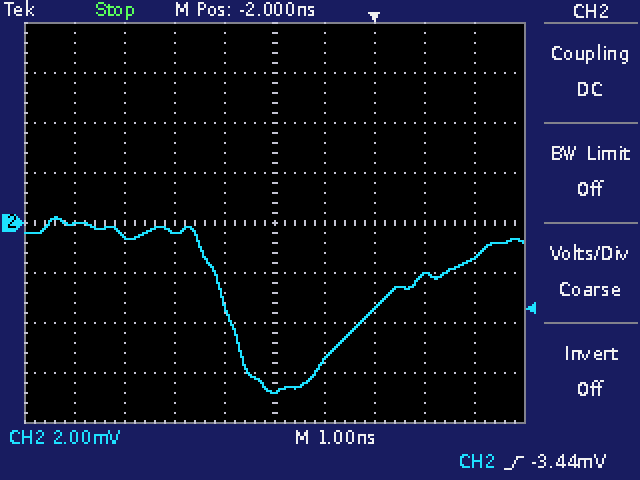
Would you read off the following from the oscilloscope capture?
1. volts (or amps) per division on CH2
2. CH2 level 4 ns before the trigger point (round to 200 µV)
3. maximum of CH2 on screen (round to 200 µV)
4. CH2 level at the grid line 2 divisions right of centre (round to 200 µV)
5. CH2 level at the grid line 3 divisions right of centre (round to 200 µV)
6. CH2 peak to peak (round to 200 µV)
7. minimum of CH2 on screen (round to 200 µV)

2 mV
-400 µV
200 µV
-3.4 mV
-2.0 mV
7.0 mV
-6.8 mV
